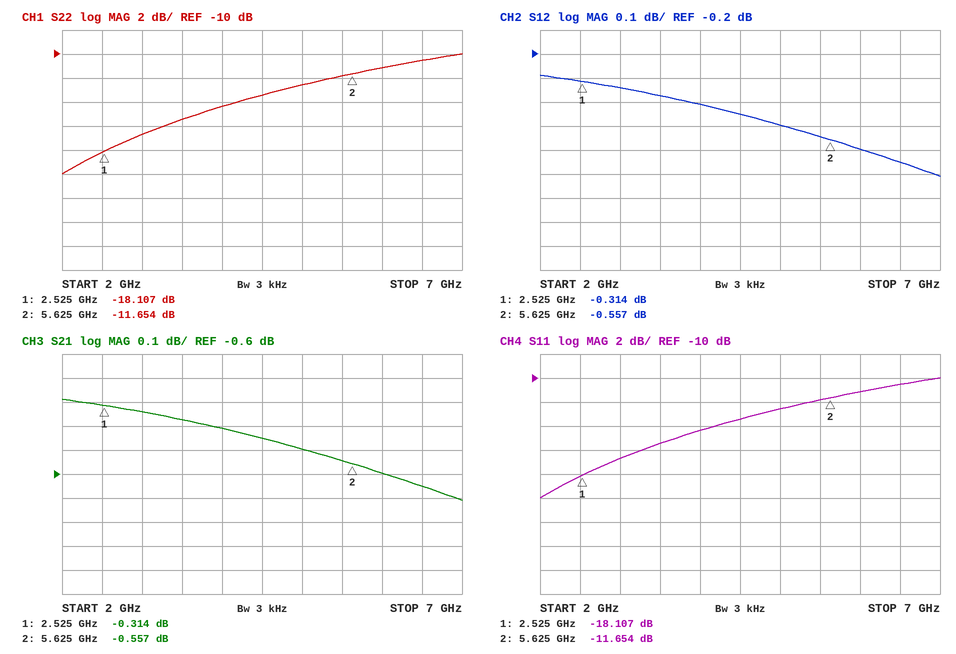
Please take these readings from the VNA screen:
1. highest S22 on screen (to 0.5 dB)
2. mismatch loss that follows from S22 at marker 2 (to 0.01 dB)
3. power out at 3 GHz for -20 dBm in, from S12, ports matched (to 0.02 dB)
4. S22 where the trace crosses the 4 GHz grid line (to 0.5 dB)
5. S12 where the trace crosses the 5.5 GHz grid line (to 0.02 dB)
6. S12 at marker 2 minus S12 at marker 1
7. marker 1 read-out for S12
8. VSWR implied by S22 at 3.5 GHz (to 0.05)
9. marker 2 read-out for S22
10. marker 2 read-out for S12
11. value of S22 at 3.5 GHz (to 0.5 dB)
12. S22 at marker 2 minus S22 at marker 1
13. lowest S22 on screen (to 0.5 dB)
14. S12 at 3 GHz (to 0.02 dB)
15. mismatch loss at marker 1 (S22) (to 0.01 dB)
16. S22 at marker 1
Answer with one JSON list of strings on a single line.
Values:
["-10.0 dB", "0.31 dB", "-20.34 dBm", "-14.5 dB", "-0.54 dB", "-0.243 dB", "-0.314 dB", "1.40", "-11.654 dB", "-0.557 dB", "-15.5 dB", "6.453 dB", "-20.0 dB", "-0.34 dB", "0.07 dB", "-18.107 dB"]
